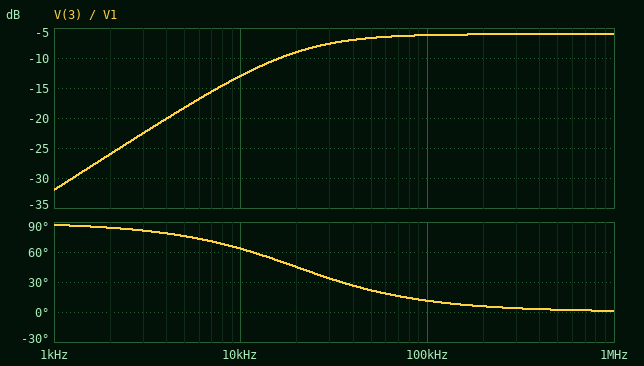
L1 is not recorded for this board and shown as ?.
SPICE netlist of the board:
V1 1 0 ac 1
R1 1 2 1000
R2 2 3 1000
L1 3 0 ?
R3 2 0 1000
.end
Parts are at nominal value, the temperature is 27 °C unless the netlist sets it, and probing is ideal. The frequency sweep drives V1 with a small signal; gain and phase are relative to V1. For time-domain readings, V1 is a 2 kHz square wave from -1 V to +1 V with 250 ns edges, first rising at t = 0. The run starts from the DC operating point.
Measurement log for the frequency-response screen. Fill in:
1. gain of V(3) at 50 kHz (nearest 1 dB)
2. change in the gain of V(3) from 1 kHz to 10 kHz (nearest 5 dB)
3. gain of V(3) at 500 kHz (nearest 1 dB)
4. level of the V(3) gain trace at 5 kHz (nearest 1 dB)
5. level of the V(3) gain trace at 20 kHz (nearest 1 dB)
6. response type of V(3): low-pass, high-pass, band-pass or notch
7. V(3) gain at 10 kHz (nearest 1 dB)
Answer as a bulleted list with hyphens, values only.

- -7 dB
- 20 dB
- -6 dB
- -18 dB
- -9 dB
- high-pass
- -13 dB
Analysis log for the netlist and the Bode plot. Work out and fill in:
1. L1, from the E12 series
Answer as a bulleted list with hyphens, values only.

- 12 mH
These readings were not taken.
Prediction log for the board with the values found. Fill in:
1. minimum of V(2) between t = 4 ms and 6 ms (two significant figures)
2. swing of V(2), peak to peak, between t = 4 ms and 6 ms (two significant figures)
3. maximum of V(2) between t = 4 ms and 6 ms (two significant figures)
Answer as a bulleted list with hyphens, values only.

- -660 mV
- 1.3 V
- 660 mV
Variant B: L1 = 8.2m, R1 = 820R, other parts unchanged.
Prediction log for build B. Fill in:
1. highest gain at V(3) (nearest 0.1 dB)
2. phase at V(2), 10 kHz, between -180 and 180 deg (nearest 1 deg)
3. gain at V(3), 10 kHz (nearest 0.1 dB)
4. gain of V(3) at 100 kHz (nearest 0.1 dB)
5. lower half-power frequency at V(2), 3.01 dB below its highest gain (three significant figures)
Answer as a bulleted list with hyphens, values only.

- -5.2 dB
- 8 deg
- -14.7 dB
- -5.5 dB
- 6.26 kHz
